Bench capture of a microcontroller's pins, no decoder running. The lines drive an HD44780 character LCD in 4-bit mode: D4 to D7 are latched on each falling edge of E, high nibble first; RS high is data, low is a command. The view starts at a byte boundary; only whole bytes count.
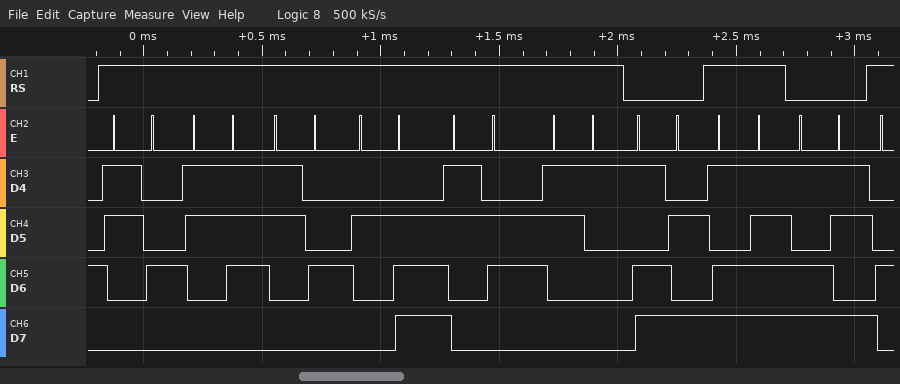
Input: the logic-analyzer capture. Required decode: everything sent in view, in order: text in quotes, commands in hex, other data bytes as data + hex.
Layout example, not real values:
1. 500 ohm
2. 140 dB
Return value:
1. "474.61" 0xDA data DF 0xDB
